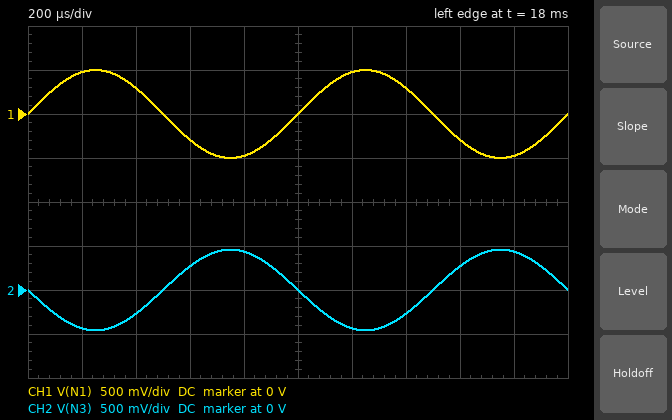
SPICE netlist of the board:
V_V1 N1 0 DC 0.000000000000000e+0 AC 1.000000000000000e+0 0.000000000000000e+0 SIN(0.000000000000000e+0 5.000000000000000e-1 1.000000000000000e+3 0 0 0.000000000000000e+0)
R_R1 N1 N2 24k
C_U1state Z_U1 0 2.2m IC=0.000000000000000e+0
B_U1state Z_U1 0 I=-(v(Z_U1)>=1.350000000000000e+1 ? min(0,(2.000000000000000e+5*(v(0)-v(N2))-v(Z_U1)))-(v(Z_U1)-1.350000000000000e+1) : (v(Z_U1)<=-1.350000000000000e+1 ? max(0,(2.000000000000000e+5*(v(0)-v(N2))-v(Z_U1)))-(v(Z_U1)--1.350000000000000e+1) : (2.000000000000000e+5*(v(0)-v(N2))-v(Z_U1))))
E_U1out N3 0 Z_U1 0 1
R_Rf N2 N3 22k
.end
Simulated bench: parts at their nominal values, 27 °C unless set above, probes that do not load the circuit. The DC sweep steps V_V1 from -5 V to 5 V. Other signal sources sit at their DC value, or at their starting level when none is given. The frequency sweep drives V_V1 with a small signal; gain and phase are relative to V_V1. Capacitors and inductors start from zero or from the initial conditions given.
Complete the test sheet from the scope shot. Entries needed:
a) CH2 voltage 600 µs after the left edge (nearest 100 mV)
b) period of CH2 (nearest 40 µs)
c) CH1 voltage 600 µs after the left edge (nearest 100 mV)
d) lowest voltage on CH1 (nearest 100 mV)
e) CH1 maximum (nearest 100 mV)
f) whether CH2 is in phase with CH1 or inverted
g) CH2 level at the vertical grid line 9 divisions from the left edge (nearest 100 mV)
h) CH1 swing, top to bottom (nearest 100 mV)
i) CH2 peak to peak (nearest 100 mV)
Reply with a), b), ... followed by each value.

a) 300 mV
b) 1.00 ms
c) -300 mV
d) -500 mV
e) 500 mV
f) inverted
g) 400 mV
h) 1.0 V
i) 900 mV
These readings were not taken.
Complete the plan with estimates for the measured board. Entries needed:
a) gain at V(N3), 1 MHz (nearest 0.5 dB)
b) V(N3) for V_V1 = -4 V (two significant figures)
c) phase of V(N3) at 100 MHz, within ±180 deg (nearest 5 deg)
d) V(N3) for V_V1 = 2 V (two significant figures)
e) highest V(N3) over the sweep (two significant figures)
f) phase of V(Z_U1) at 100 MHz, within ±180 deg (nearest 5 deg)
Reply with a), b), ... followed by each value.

a) -1.0 dB
b) 3.7 V
c) 95 deg
d) -1.8 V
e) 4.6 V
f) 95 deg
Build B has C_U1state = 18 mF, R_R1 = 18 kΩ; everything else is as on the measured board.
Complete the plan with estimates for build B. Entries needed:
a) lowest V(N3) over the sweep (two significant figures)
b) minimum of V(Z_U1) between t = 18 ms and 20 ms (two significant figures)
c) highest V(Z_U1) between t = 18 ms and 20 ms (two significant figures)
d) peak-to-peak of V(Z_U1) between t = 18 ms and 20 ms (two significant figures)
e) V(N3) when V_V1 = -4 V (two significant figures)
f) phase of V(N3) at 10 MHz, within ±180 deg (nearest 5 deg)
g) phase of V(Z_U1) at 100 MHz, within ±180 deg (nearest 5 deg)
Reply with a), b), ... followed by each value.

a) -6.1 V
b) -610 mV
c) 610 mV
d) 1.2 V
e) 4.9 V
f) 95 deg
g) 90 deg
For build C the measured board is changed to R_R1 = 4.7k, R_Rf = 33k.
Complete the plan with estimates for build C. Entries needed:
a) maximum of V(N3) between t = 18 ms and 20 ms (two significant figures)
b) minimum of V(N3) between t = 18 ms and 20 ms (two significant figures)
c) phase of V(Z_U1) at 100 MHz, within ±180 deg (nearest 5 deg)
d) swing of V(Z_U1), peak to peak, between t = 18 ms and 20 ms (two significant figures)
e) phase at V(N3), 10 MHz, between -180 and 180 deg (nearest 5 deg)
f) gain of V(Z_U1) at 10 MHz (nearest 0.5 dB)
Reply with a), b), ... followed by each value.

a) 3.5 V
b) -3.5 V
c) 90 deg
d) 7.0 V
e) 100 deg
f) 2.0 dB
